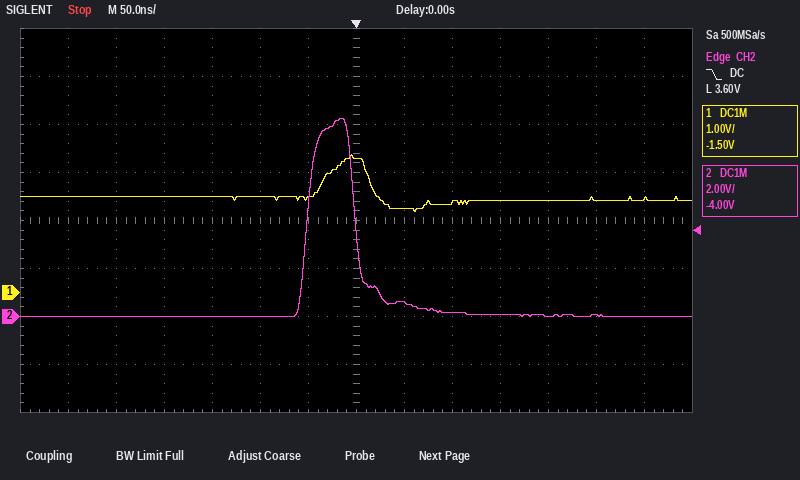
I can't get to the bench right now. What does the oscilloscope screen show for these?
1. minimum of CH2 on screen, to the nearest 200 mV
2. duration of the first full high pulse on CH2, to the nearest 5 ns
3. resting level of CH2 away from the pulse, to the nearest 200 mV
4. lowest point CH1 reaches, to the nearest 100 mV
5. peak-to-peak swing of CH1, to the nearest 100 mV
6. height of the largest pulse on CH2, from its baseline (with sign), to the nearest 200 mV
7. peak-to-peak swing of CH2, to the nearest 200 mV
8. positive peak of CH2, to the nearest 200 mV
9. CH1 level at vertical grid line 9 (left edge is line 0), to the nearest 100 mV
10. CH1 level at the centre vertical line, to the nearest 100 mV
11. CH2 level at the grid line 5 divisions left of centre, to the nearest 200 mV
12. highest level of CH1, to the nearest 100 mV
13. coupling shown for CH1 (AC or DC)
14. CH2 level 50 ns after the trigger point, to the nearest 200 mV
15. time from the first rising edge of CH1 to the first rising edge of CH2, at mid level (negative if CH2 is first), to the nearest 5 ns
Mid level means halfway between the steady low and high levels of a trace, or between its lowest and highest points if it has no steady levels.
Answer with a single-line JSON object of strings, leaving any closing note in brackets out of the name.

{"minimum of CH2 on screen, to the nearest 200 mV": "0.0 V", "duration of the first full high pulse on CH2, to the nearest 5 ns": "50 ns", "resting level of CH2 away from the pulse, to the nearest 200 mV": "0.0 V", "lowest point CH1 reaches, to the nearest 100 mV": "1.7 V", "peak-to-peak swing of CH1, to the nearest 100 mV": "1.2 V", "height of the largest pulse on CH2, from its baseline (with sign), to the nearest 200 mV": "+8.2 V", "peak-to-peak swing of CH2, to the nearest 200 mV": "8.2 V", "positive peak of CH2, to the nearest 200 mV": "8.2 V", "CH1 level at vertical grid line 9 (left edge is line 0), to the nearest 100 mV": "1.9 V", "CH1 level at the centre vertical line, to the nearest 100 mV": "2.8 V", "CH2 level at the grid line 5 divisions left of centre, to the nearest 200 mV": "0.0 V", "highest level of CH1, to the nearest 100 mV": "2.9 V", "coupling shown for CH1": "DC", "CH2 level 50 ns after the trigger point, to the nearest 200 mV": "600 mV", "time from the first rising edge of CH1 to the first rising edge of CH2, at mid level (negative if CH2 is first), to the nearest 5 ns": "-15 ns"}
